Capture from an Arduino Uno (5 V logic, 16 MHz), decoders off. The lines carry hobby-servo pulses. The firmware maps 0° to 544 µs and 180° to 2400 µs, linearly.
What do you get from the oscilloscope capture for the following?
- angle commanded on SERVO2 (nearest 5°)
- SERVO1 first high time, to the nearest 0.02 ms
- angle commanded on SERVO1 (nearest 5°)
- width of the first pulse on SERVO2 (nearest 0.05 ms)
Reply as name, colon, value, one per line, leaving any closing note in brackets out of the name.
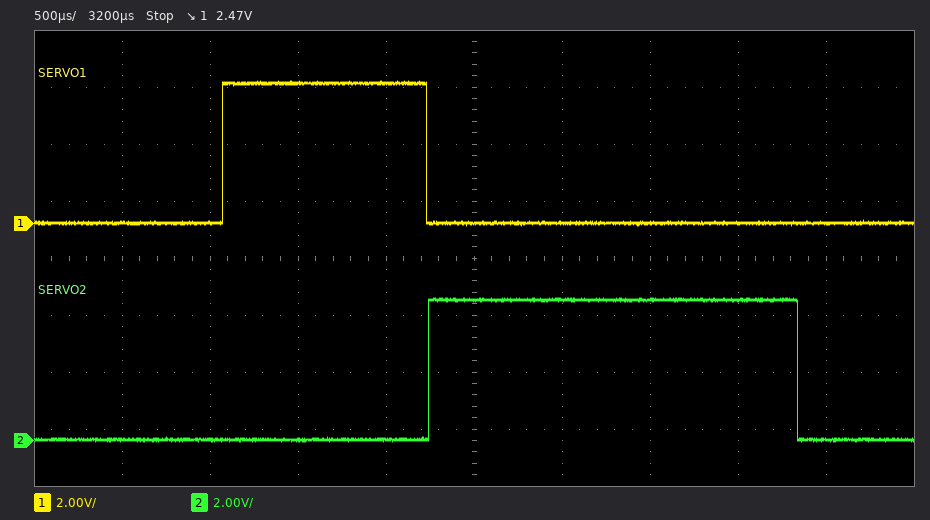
angle commanded on SERVO2: 150°
SERVO1 first high time, to the nearest 0.02 ms: 1.16 ms
angle commanded on SERVO1: 60°
width of the first pulse on SERVO2: 2.10 ms
